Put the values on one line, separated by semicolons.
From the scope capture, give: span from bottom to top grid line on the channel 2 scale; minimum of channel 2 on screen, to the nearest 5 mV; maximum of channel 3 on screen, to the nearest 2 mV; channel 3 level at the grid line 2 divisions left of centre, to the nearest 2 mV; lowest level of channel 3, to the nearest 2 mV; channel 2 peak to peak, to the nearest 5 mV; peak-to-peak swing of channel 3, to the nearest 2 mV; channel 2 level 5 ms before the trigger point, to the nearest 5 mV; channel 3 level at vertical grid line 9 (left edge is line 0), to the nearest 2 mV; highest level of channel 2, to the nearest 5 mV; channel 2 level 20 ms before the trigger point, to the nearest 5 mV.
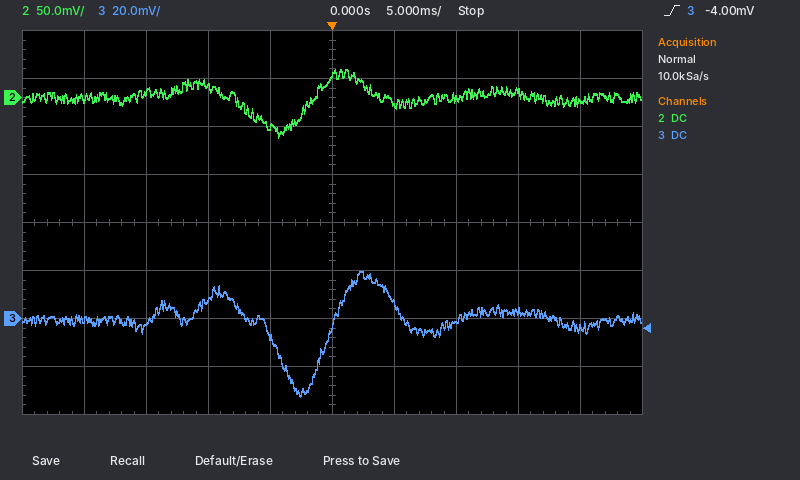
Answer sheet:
400 mV; -40 mV; 20 mV; 8 mV; -32 mV; 70 mV; 52 mV; -30 mV; -4 mV; 30 mV; 0 mV
